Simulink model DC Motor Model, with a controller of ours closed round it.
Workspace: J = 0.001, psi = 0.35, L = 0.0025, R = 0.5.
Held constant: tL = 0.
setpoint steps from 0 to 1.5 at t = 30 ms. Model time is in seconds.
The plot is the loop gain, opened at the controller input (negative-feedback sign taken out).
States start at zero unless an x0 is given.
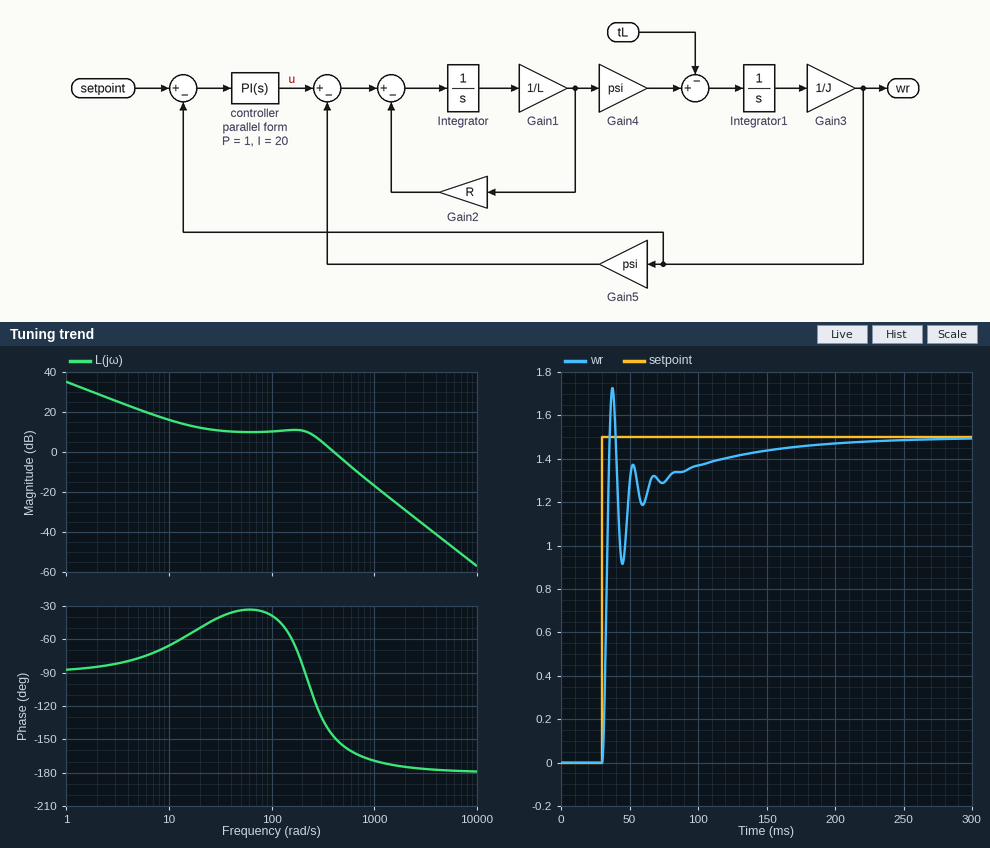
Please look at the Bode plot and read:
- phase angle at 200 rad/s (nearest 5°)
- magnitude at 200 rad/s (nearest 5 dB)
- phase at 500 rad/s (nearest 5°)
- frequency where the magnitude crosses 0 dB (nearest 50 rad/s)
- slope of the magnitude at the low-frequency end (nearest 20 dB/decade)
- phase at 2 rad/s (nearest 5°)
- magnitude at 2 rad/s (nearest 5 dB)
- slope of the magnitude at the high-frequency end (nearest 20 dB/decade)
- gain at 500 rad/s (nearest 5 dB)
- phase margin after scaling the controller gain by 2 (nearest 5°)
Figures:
-85°
10 dB
-155°
400 rad/s
-20 dB/decade
-85°
30 dB
-40 dB/decade
-5 dB
20°
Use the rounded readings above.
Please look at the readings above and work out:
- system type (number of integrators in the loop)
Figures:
1
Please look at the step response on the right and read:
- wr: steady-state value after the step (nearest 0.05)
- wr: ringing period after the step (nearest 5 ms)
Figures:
1.50
15 ms
